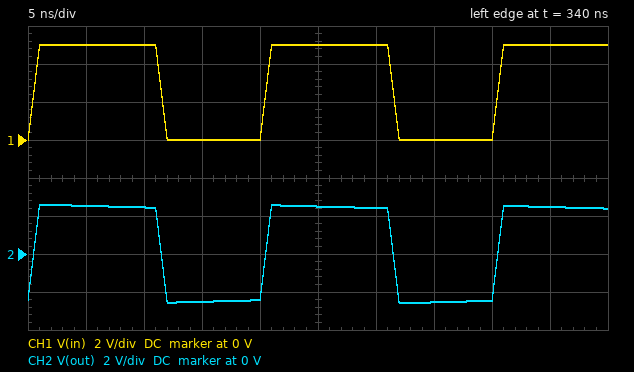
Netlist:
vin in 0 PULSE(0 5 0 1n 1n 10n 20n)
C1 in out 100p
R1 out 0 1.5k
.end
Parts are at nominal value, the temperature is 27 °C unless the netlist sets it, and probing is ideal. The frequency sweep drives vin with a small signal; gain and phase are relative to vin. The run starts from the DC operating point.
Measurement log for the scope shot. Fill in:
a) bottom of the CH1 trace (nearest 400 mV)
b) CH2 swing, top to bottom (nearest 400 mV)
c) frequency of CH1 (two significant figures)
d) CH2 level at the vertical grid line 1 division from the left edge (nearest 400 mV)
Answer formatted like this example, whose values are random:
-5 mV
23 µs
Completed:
0 V
5.2 V
50 MHz
2.4 V
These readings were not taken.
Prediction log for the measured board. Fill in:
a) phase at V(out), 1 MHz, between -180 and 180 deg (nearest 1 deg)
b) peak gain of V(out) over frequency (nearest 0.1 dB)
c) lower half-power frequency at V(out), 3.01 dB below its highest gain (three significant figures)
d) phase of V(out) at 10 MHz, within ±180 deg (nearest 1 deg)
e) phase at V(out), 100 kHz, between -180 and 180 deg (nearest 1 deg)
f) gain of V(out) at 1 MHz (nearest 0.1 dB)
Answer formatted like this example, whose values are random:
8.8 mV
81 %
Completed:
47 deg
0 dB
1.06 MHz
6 deg
85 deg
-3.3 dB
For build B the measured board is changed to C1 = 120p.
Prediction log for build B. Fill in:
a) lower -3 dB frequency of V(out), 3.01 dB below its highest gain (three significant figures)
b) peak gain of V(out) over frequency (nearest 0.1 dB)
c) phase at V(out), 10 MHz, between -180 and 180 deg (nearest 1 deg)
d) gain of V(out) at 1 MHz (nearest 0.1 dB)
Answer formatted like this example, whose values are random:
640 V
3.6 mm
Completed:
884 kHz
0 dB
5 deg
-2.5 dB
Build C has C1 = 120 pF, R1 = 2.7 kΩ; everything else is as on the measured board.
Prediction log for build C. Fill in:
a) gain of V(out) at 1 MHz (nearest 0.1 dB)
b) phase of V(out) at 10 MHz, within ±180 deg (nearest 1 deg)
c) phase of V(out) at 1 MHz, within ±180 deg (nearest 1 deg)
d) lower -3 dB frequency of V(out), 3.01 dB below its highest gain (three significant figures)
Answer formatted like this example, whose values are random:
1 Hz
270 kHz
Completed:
-0.9 dB
3 deg
26 deg
491 kHz
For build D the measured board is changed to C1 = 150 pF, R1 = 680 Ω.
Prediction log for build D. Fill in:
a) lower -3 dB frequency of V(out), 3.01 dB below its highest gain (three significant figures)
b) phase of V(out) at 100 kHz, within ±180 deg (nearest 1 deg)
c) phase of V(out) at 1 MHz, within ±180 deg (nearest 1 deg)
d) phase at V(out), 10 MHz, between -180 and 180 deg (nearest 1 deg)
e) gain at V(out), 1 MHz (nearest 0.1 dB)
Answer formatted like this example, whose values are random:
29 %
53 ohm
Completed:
1.56 MHz
86 deg
57 deg
9 deg
-5.4 dB
